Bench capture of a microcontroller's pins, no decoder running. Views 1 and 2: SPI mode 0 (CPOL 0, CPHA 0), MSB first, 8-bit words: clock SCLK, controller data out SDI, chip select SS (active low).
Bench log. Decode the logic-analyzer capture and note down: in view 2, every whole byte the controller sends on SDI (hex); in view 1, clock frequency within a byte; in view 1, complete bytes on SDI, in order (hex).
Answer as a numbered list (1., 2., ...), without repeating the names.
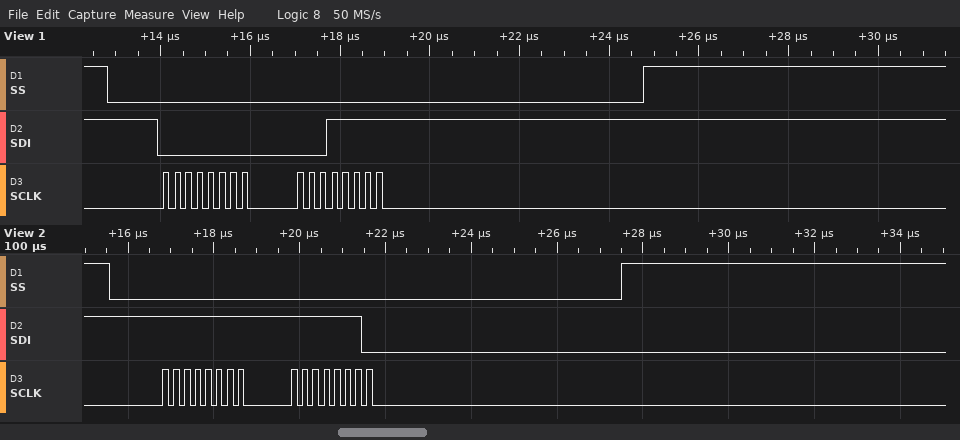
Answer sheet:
1. FF FE
2. 4 MHz
3. 00 1F
